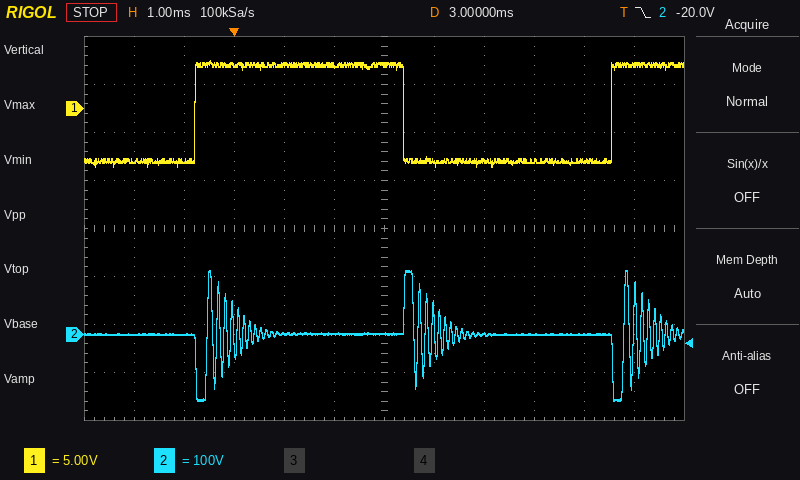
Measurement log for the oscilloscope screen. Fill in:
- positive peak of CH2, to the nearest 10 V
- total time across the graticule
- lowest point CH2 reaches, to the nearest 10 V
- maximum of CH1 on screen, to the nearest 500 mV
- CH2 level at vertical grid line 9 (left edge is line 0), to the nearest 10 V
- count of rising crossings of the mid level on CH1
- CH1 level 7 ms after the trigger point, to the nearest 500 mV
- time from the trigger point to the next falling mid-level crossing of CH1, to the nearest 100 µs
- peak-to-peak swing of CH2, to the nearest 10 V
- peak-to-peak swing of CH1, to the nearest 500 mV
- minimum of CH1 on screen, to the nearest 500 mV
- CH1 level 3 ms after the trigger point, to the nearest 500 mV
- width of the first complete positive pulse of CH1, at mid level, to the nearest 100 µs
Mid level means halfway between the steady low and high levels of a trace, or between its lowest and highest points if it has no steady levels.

130 V
12 ms
-140 V
5.0 V
0 V
2
-5.5 V
3.4 ms
270 V
11.0 V
-6.0 V
4.5 V
4.2 ms
